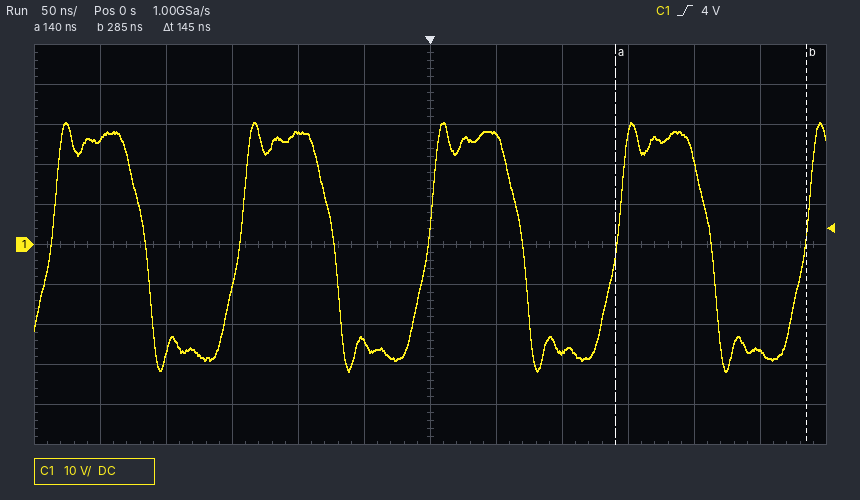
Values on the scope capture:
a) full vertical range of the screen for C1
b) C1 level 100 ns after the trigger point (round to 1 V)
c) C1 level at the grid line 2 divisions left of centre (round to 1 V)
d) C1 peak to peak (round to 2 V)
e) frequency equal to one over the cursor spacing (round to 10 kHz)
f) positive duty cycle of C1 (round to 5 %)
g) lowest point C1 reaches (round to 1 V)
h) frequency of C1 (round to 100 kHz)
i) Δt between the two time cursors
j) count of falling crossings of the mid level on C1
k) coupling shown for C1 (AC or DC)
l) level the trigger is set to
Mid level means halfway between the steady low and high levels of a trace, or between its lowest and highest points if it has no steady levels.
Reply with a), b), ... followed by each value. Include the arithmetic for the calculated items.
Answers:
a) 100 V
b) -27 V
c) 28 V
d) 62 V
e) 1 / 145 ns ≈ 6.90 MHz
f) 50 %
g) -32 V
h) 7.0 MHz
i) 145 ns
j) 4
k) DC
l) 4 V
